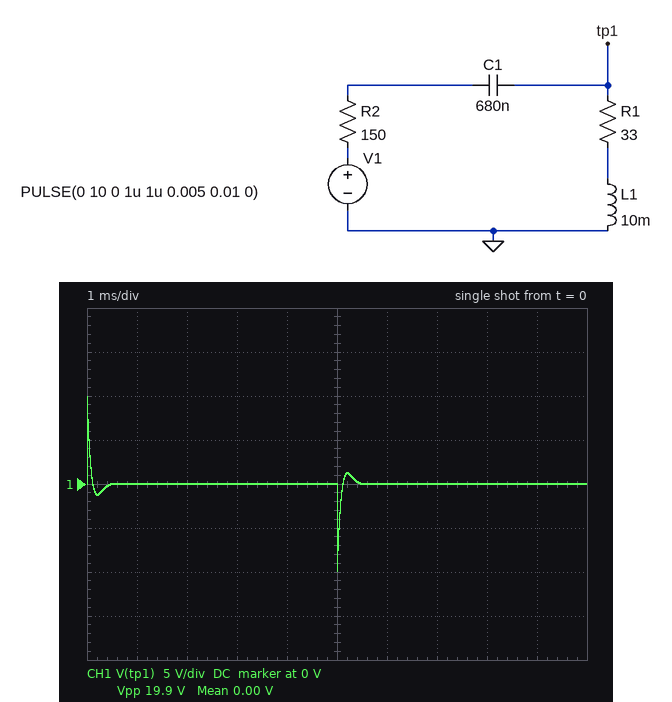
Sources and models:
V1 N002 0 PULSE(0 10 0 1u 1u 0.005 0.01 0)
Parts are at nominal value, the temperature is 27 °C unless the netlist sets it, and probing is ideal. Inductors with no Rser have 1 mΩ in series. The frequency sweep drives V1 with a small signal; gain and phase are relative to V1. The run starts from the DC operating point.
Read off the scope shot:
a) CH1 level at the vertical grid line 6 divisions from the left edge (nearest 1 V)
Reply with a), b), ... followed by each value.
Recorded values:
a) 0 V
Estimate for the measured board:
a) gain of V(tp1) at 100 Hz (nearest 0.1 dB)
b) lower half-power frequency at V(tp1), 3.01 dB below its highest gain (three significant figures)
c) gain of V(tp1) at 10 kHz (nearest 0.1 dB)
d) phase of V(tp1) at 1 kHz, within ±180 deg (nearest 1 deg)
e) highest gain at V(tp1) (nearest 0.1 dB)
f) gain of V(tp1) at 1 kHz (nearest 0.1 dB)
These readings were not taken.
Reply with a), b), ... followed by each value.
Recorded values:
a) -36.9 dB
b) 1.99 kHz
c) 0 dB
d) 105 deg
e) 0 dB
f) -11.0 dB
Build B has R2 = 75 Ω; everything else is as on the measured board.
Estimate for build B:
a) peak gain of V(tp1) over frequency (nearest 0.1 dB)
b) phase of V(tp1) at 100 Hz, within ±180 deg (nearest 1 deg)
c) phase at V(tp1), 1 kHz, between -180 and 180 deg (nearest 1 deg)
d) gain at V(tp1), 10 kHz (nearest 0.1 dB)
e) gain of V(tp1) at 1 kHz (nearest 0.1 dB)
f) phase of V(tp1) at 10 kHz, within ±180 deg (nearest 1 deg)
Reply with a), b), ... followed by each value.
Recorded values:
a) 2.2 dB
b) 98 deg
c) 120 deg
d) 0.2 dB
e) -9.1 dB
f) 7 deg
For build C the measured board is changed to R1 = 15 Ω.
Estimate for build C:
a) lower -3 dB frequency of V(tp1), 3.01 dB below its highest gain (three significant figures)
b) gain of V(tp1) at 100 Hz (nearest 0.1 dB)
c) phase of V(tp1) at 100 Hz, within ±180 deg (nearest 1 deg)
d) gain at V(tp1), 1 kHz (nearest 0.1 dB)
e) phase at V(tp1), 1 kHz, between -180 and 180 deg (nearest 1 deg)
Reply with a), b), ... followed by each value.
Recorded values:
a) 1.85 kHz
b) -43.2 dB
c) 109 deg
d) -11.3 dB
e) 123 deg
